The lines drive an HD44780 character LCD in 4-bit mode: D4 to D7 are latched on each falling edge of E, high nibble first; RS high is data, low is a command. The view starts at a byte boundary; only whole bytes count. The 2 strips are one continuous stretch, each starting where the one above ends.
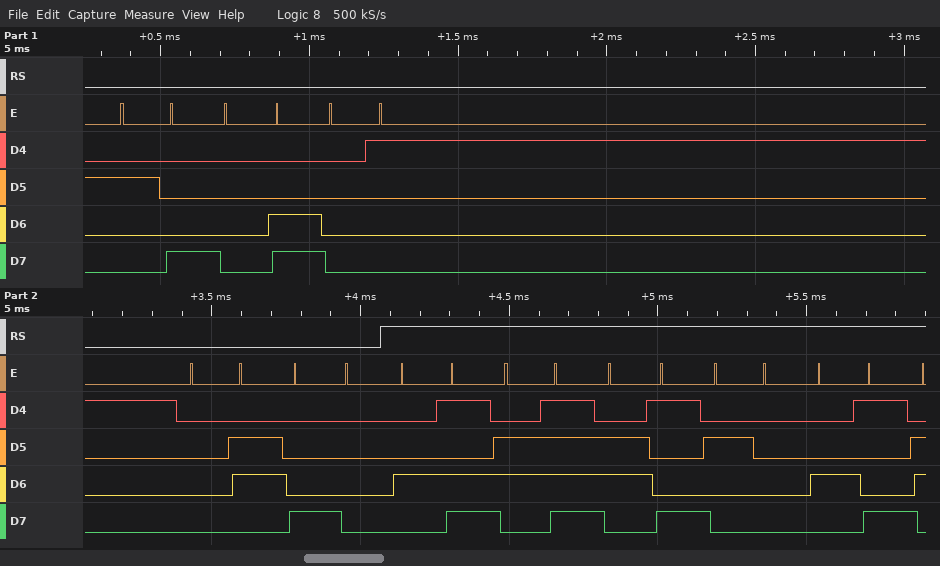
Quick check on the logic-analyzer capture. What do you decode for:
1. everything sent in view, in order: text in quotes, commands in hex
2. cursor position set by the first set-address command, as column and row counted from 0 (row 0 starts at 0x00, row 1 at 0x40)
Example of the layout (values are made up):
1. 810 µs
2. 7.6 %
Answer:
1. 0x28 0x0C 0x01 0x06 0x80 "Moi I"
2. column 0, row 0
